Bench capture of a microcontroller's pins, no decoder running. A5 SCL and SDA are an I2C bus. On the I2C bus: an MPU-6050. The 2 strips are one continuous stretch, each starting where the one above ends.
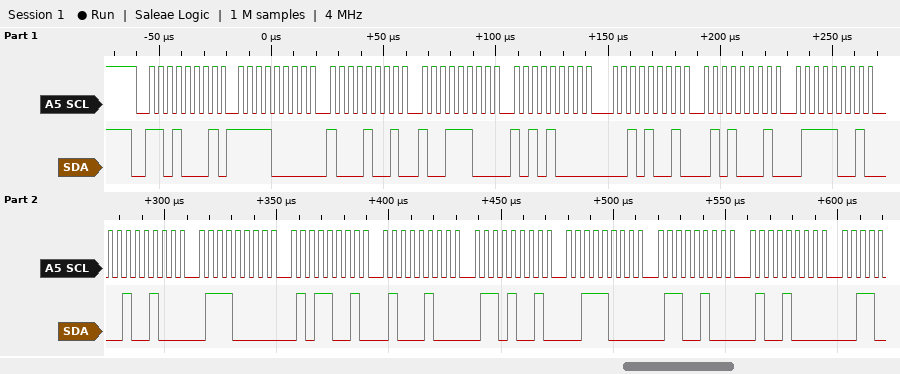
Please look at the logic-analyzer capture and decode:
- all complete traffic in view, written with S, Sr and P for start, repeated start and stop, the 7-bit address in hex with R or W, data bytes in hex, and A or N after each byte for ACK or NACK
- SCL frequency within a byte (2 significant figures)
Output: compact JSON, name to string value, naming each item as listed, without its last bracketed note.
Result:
{"all complete traffic in view, written with S, Sr and P for start, repeated start and stop, the 7-bit address in hex with R or W, data bytes in hex, and A or N after each byte for ACK or NACK": "S 68R A F0 A 89 A 9C A A8 A 29 A 51 A 79 A 24 A 70 A 59 A 44 A 69 A 38 A 64 A 48 A", "SCL frequency within a byte": "250 kHz"}
